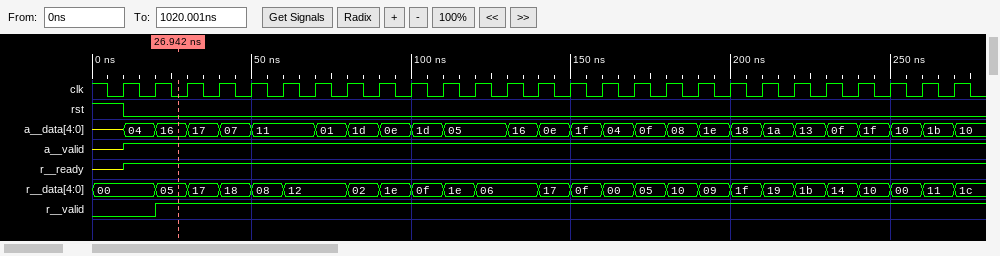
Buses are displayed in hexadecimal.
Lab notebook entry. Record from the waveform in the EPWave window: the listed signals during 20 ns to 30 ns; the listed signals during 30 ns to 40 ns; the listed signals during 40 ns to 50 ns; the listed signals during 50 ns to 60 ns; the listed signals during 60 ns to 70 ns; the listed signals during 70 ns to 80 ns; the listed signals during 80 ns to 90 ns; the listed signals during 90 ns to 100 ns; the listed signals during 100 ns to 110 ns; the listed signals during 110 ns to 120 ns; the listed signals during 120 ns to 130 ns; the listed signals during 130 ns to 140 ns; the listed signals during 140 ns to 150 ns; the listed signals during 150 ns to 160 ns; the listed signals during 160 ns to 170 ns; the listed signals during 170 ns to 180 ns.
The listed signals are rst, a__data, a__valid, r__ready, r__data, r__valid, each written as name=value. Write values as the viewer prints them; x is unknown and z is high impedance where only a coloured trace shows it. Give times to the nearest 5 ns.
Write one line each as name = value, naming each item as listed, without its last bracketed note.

the listed signals during 20 ns to 30 ns = rst=0, a__data=16, a__valid=1, r__ready=1, r__data=05, r__valid=1
the listed signals during 30 ns to 40 ns = rst=0, a__data=17, a__valid=1, r__ready=1, r__data=17, r__valid=1
the listed signals during 40 ns to 50 ns = rst=0, a__data=07, a__valid=1, r__ready=1, r__data=18, r__valid=1
the listed signals during 50 ns to 60 ns = rst=0, a__data=11, a__valid=1, r__ready=1, r__data=08, r__valid=1
the listed signals during 60 ns to 70 ns = rst=0, a__data=11, a__valid=1, r__ready=1, r__data=12, r__valid=1
the listed signals during 70 ns to 80 ns = rst=0, a__data=01, a__valid=1, r__ready=1, r__data=12, r__valid=1
the listed signals during 80 ns to 90 ns = rst=0, a__data=1d, a__valid=1, r__ready=1, r__data=02, r__valid=1
the listed signals during 90 ns to 100 ns = rst=0, a__data=0e, a__valid=1, r__ready=1, r__data=1e, r__valid=1
the listed signals during 100 ns to 110 ns = rst=0, a__data=1d, a__valid=1, r__ready=1, r__data=0f, r__valid=1
the listed signals during 110 ns to 120 ns = rst=0, a__data=05, a__valid=1, r__ready=1, r__data=1e, r__valid=1
the listed signals during 120 ns to 130 ns = rst=0, a__data=05, a__valid=1, r__ready=1, r__data=06, r__valid=1
the listed signals during 130 ns to 140 ns = rst=0, a__data=16, a__valid=1, r__ready=1, r__data=06, r__valid=1
the listed signals during 140 ns to 150 ns = rst=0, a__data=0e, a__valid=1, r__ready=1, r__data=17, r__valid=1
the listed signals during 150 ns to 160 ns = rst=0, a__data=1f, a__valid=1, r__ready=1, r__data=0f, r__valid=1
the listed signals during 160 ns to 170 ns = rst=0, a__data=04, a__valid=1, r__ready=1, r__data=00, r__valid=1
the listed signals during 170 ns to 180 ns = rst=0, a__data=0f, a__valid=1, r__ready=1, r__data=05, r__valid=1
